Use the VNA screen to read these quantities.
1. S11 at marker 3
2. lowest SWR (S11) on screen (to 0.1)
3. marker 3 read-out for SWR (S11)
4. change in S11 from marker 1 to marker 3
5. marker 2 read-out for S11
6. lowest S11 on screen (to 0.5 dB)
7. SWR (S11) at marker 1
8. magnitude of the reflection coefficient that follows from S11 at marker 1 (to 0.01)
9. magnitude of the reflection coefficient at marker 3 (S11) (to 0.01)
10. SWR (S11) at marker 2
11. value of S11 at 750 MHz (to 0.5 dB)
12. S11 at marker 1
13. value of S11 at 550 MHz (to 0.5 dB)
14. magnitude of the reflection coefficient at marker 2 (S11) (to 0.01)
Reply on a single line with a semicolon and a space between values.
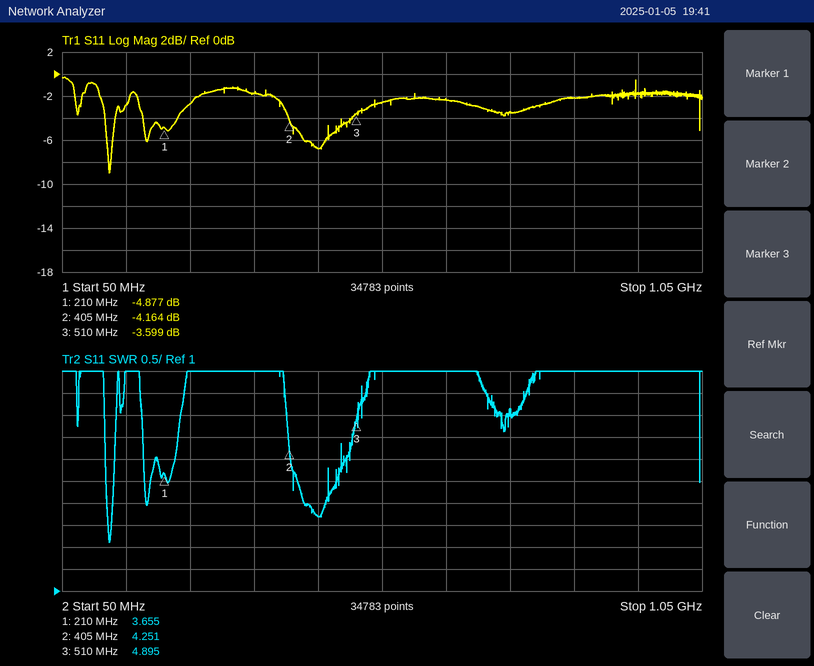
-3.599 dB; 2.1; 4.895; 1.278 dB; -4.164 dB; -9.0 dB; 3.655; 0.57; 0.66; 4.251; -3.5 dB; -4.877 dB; -2.5 dB; 0.62
